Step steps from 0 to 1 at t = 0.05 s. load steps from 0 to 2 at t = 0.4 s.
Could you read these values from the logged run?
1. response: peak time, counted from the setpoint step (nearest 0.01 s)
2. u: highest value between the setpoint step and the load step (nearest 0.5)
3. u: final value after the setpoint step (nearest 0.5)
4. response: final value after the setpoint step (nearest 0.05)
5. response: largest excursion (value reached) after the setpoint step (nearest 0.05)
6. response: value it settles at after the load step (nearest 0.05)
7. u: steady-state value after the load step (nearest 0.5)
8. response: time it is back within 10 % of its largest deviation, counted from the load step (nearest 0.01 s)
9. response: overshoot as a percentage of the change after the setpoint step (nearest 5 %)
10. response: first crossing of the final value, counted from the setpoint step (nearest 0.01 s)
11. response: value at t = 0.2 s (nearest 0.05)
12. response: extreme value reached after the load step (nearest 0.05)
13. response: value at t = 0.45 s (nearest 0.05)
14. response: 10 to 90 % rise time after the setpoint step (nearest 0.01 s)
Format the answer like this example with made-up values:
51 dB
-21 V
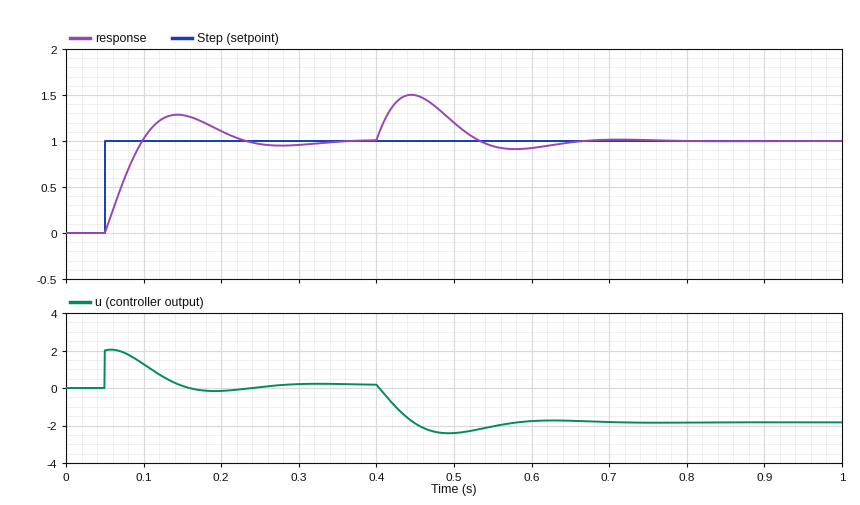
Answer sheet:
0.09 s
2.0
0.0
1.00
1.30
1.00
-2.0
0.22 s
30 %
0.05 s
1.10
1.50
1.50
0.04 s
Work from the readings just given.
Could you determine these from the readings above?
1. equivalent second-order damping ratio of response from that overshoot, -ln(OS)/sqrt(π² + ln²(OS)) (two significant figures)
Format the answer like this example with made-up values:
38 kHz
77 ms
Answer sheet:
0.36
